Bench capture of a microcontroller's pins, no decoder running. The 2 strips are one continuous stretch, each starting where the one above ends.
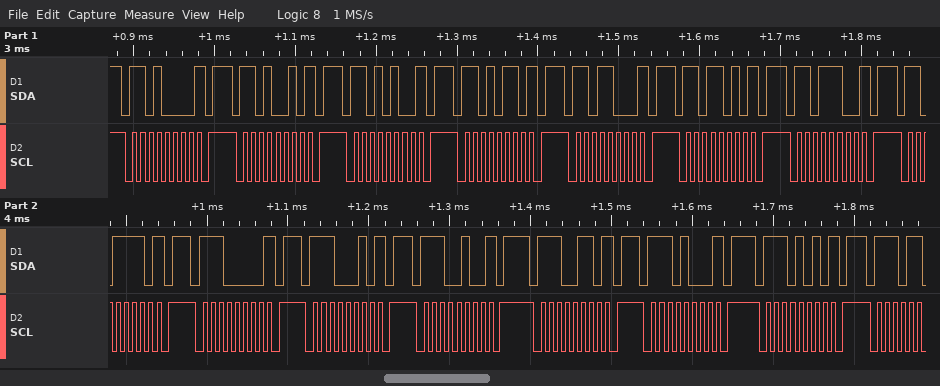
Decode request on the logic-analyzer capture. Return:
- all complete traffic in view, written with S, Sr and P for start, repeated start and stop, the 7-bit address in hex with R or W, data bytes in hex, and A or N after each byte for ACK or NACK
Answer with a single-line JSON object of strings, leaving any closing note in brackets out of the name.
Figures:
{"all complete traffic in view, written with S, Sr and P for start, repeated start and stop, the 7-bit address in hex with R or W, data bytes in hex, and A or N after each byte for ACK or NACK": "S 68W N P S 69W N P S 6AW N P S 6BW N P S 6CW N P S 6DW N P S 6EW N P S 6FW N P S 70W N P S 71W N P S 72W N P S 73W N P S 74W N P S 75W N P"}
